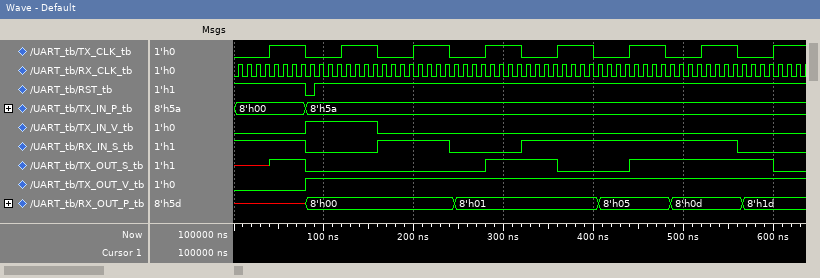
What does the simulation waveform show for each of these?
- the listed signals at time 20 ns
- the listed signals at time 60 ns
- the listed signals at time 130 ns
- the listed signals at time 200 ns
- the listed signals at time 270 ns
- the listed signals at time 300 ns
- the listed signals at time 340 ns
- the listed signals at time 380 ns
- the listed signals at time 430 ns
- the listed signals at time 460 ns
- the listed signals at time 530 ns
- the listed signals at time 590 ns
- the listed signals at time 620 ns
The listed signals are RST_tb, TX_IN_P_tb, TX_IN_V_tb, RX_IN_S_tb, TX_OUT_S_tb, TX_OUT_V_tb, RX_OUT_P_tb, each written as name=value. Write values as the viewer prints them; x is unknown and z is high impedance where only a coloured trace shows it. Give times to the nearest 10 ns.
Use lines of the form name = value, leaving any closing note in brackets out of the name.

the listed signals at time 20 ns = RST_tb=1, TX_IN_P_tb=8'h00, TX_IN_V_tb=0, RX_IN_S_tb=1, TX_OUT_S_tb=x, TX_OUT_V_tb=0, RX_OUT_P_tb=x
the listed signals at time 60 ns = RST_tb=1, TX_IN_P_tb=8'h00, TX_IN_V_tb=0, RX_IN_S_tb=1, TX_OUT_S_tb=1, TX_OUT_V_tb=0, RX_OUT_P_tb=x
the listed signals at time 130 ns = RST_tb=1, TX_IN_P_tb=8'h5a, TX_IN_V_tb=1, RX_IN_S_tb=0, TX_OUT_S_tb=0, TX_OUT_V_tb=1, RX_OUT_P_tb=8'h00
the listed signals at time 200 ns = RST_tb=1, TX_IN_P_tb=8'h5a, TX_IN_V_tb=0, RX_IN_S_tb=1, TX_OUT_S_tb=0, TX_OUT_V_tb=1, RX_OUT_P_tb=8'h00
the listed signals at time 270 ns = RST_tb=1, TX_IN_P_tb=8'h5a, TX_IN_V_tb=0, RX_IN_S_tb=0, TX_OUT_S_tb=0, TX_OUT_V_tb=1, RX_OUT_P_tb=8'h01
the listed signals at time 300 ns = RST_tb=1, TX_IN_P_tb=8'h5a, TX_IN_V_tb=0, RX_IN_S_tb=0, TX_OUT_S_tb=1, TX_OUT_V_tb=1, RX_OUT_P_tb=8'h01
the listed signals at time 340 ns = RST_tb=1, TX_IN_P_tb=8'h5a, TX_IN_V_tb=0, RX_IN_S_tb=1, TX_OUT_S_tb=1, TX_OUT_V_tb=1, RX_OUT_P_tb=8'h01
the listed signals at time 380 ns = RST_tb=1, TX_IN_P_tb=8'h5a, TX_IN_V_tb=0, RX_IN_S_tb=1, TX_OUT_S_tb=0, TX_OUT_V_tb=1, RX_OUT_P_tb=8'h01
the listed signals at time 430 ns = RST_tb=1, TX_IN_P_tb=8'h5a, TX_IN_V_tb=0, RX_IN_S_tb=1, TX_OUT_S_tb=0, TX_OUT_V_tb=1, RX_OUT_P_tb=8'h05
the listed signals at time 460 ns = RST_tb=1, TX_IN_P_tb=8'h5a, TX_IN_V_tb=0, RX_IN_S_tb=1, TX_OUT_S_tb=1, TX_OUT_V_tb=1, RX_OUT_P_tb=8'h05
the listed signals at time 530 ns = RST_tb=1, TX_IN_P_tb=8'h5a, TX_IN_V_tb=0, RX_IN_S_tb=1, TX_OUT_S_tb=1, TX_OUT_V_tb=1, RX_OUT_P_tb=8'h0d
the listed signals at time 590 ns = RST_tb=1, TX_IN_P_tb=8'h5a, TX_IN_V_tb=0, RX_IN_S_tb=0, TX_OUT_S_tb=1, TX_OUT_V_tb=1, RX_OUT_P_tb=8'h1d
the listed signals at time 620 ns = RST_tb=1, TX_IN_P_tb=8'h5a, TX_IN_V_tb=0, RX_IN_S_tb=0, TX_OUT_S_tb=0, TX_OUT_V_tb=1, RX_OUT_P_tb=8'h1d
